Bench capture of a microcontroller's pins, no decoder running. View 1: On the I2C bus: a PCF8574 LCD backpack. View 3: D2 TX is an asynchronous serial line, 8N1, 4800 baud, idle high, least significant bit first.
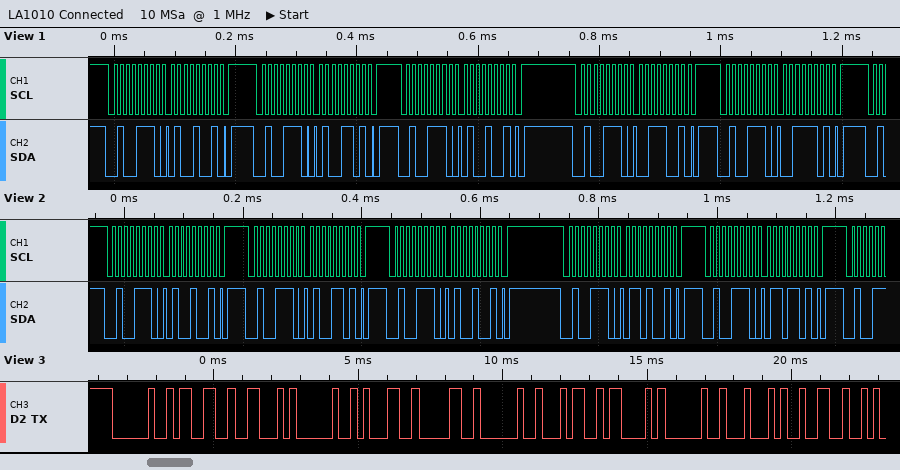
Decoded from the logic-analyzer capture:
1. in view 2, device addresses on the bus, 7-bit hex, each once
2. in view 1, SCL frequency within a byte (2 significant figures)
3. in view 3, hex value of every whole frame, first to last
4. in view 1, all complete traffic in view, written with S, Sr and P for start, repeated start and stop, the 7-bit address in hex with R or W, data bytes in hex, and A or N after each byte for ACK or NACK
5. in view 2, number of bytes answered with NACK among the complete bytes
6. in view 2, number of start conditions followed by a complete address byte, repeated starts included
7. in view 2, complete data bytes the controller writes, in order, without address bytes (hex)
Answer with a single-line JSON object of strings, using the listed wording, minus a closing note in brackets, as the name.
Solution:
{"in view 2, device addresses on the bus, 7-bit hex, each once": "0x27", "in view 1, SCL frequency within a byte": "100 kHz", "in view 3, hex value of every whole frame, first to last": "0x20 0x33 0x46 0x20 0x31 0x30 0x20 0x34 0x43 0x20 0x44 0x32", "in view 1, all complete traffic in view, written with S, Sr and P for start, repeated start and stop, the 7-bit address in hex with R or W, data bytes in hex, and A or N after each byte for ACK or NACK": "S 27W A 49 A P S 27W A 4D A P S 27W A 49 A P S 27W A 39 A P S 27W A 3D A P", "in view 2, number of bytes answered with NACK among the complete bytes": "0", "in view 2, number of start conditions followed by a complete address byte, repeated starts included": "5", "in view 2, complete data bytes the controller writes, in order, without address bytes": "49 4D 49 69 6D"}
